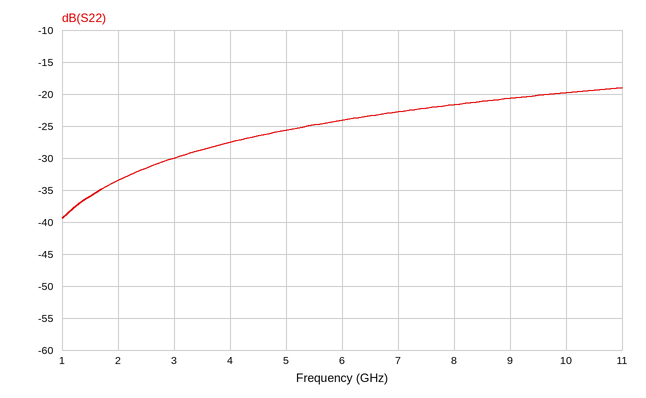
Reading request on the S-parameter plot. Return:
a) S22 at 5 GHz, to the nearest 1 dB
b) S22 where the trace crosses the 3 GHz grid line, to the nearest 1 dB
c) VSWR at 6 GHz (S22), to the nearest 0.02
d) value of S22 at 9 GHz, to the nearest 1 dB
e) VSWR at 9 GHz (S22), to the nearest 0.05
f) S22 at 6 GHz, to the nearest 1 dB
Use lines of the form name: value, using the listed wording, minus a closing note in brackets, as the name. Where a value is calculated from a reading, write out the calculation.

S22 at 5 GHz, to the nearest 1 dB: -26 dB
S22 where the trace crosses the 3 GHz grid line, to the nearest 1 dB: -30 dB
VSWR at 6 GHz (S22), to the nearest 0.02: |Γ| = 10^(-24/20) = 0.0631; VSWR = (1 + 0.0631)/(1 − 0.0631) ≈ 1.13, so 1.14 to the nearest 0.02
value of S22 at 9 GHz, to the nearest 1 dB: -21 dB
VSWR at 9 GHz (S22), to the nearest 0.05: |Γ| = 10^(-21/20) = 0.0891; VSWR = (1 + 0.0891)/(1 − 0.0891) ≈ 1.20
S22 at 6 GHz, to the nearest 1 dB: -24 dB
